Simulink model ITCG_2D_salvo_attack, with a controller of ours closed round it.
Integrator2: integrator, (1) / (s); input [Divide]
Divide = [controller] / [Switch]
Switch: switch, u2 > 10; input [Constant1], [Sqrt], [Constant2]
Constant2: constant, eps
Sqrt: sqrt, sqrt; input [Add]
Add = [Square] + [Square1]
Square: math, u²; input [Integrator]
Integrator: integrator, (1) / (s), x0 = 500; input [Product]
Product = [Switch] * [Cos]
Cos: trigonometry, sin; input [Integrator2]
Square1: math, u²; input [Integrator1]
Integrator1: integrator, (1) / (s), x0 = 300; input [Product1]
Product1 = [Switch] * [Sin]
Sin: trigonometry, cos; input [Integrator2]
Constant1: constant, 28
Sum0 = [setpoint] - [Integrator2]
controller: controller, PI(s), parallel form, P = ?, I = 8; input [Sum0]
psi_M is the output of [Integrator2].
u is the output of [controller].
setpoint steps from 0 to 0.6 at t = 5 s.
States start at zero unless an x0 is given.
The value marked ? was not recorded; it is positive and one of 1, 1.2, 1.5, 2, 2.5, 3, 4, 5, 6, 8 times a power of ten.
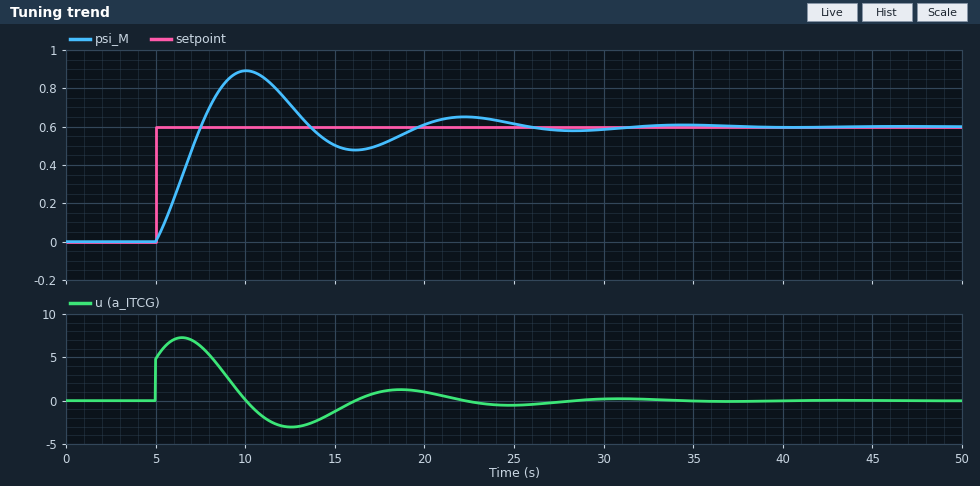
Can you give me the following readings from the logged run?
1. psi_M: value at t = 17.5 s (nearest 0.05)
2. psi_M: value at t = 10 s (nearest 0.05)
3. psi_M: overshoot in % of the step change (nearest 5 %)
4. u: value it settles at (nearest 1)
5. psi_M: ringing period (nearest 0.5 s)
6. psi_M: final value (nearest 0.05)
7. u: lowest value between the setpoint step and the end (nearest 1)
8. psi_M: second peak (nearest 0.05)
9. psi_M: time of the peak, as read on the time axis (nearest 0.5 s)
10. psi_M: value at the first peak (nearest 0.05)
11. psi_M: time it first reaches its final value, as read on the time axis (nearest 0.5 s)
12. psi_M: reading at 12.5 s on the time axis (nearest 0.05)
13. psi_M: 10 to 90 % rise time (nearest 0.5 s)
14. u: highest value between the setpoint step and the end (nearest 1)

0.50
0.90
50 %
0
12.0 s
0.60
-3
0.65
10.0 s
0.90
7.5 s
0.70
2.0 s
7
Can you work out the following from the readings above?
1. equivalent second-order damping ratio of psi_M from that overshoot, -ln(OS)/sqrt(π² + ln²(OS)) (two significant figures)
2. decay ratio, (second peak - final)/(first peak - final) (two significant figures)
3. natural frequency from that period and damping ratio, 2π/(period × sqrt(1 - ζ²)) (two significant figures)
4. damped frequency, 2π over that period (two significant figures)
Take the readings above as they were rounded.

0.22
0.17
0.54 rad/s
0.52 rad/s
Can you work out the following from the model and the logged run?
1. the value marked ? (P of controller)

8
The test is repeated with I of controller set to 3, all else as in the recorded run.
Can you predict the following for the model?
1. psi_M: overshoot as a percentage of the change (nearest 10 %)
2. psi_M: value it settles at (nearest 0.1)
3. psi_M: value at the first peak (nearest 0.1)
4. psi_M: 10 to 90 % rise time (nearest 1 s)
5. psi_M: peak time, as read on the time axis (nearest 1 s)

30 %
0.6
0.8
3 s
13 s
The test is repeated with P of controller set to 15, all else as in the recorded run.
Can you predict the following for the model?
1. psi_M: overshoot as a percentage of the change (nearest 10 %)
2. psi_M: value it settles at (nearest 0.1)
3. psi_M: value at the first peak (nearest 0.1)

30 %
0.6
0.8
